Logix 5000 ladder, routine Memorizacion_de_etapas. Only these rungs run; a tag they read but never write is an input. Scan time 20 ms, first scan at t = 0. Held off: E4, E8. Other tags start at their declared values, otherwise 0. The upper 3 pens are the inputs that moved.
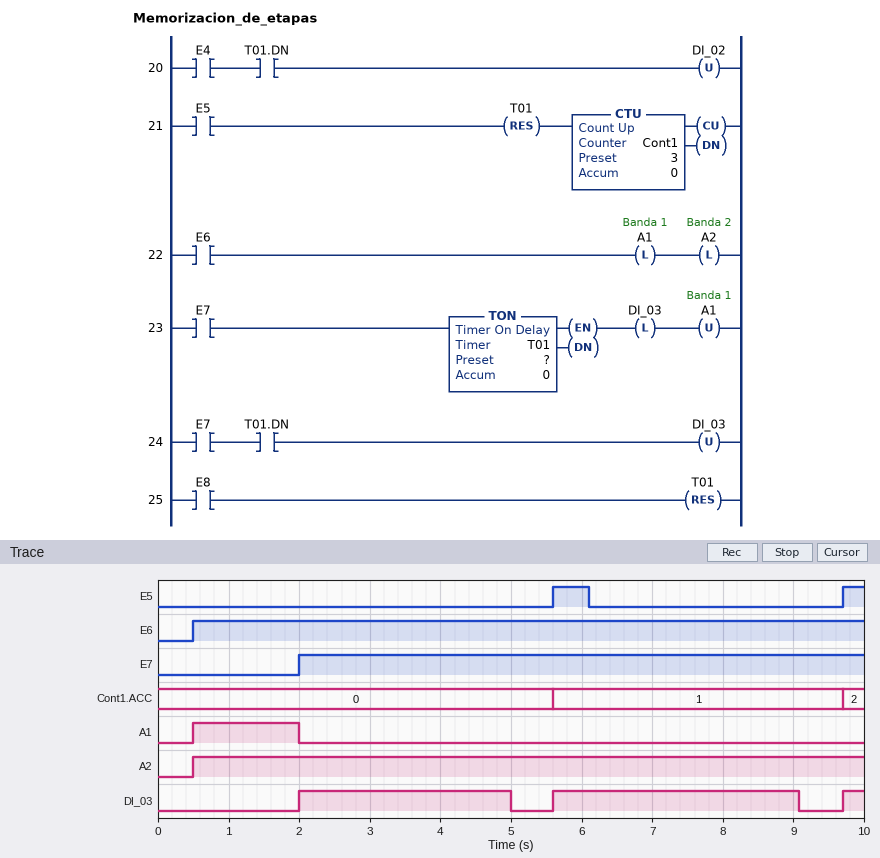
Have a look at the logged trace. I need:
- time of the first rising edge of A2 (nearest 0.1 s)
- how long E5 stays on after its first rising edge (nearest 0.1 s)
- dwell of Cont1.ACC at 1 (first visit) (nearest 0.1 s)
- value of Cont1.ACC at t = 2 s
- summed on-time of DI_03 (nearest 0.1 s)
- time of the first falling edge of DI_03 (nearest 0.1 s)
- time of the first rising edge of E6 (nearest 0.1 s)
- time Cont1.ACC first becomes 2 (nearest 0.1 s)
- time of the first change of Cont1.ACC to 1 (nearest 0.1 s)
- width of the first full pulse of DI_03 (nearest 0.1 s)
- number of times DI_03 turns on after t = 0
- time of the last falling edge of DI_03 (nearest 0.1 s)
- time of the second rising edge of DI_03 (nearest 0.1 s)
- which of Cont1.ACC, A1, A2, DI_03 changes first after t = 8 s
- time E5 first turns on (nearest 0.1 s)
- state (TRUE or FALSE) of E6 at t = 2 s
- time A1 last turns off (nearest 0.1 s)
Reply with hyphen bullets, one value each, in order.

- 0.5 s
- 0.5 s
- 4.1 s
- 0
- 6.8 s
- 5.0 s
- 0.5 s
- 9.7 s
- 5.6 s
- 3.0 s
- 3
- 9.1 s
- 5.6 s
- DI_03
- 5.6 s
- TRUE
- 2.0 s
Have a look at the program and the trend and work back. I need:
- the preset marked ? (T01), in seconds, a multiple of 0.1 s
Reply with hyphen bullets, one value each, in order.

- 3.0 s
